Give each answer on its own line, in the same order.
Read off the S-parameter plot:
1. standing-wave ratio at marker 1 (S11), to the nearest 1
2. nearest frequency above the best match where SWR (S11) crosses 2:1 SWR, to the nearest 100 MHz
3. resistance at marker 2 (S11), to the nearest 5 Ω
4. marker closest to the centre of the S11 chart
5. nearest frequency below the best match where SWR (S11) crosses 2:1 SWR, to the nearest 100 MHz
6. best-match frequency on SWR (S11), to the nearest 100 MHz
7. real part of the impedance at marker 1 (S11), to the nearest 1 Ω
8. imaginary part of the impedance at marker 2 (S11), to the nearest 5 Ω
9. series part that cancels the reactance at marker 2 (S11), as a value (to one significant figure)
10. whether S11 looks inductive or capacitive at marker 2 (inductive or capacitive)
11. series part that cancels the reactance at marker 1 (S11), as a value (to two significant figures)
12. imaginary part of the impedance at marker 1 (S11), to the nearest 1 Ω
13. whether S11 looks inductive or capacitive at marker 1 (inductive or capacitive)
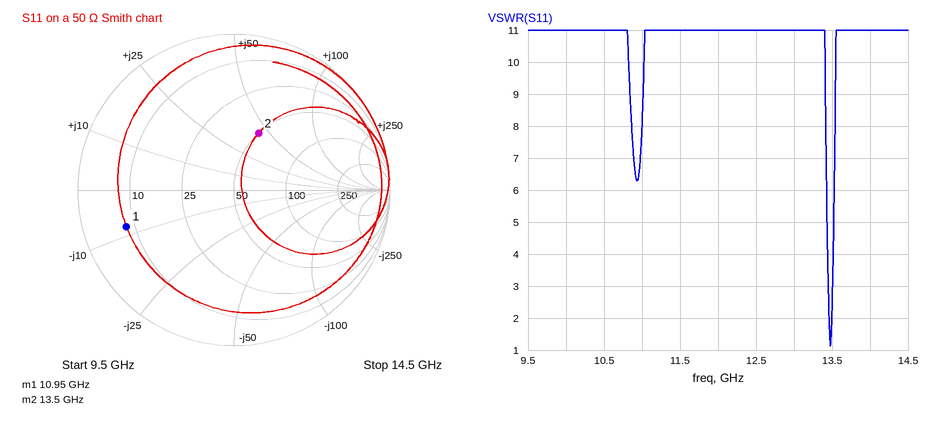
6
13.5 GHz
50 Ω
marker 2
13.5 GHz
13.5 GHz
8 Ω
+45 Ω
300 fF
inductive
120 pH
-8 Ω
capacitive
